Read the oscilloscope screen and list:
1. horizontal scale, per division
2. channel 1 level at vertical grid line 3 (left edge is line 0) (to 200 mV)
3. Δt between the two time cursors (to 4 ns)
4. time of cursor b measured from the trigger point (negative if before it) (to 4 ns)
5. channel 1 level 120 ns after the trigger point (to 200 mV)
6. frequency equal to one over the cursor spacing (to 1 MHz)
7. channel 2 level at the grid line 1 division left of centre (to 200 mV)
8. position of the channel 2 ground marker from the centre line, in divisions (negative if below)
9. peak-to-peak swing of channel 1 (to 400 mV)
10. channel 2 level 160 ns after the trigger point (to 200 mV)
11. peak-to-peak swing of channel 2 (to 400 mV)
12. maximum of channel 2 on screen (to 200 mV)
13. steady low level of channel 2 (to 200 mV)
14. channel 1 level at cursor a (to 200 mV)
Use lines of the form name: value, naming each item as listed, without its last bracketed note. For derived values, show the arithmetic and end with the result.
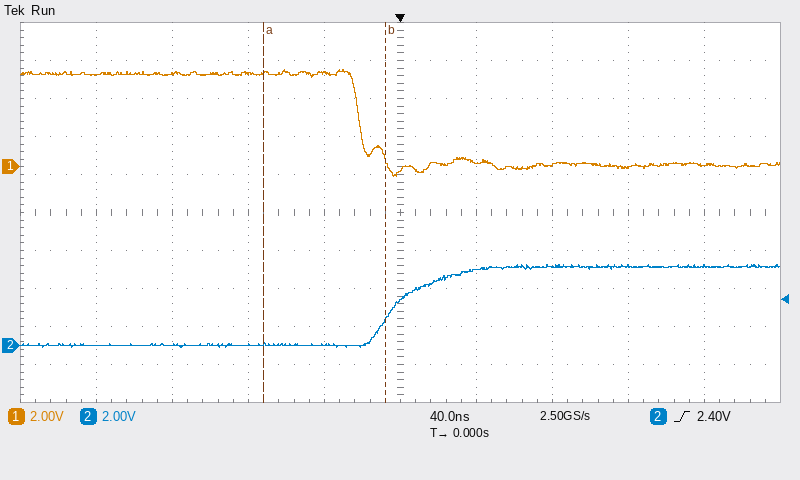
horizontal scale, per division: 40 ns
channel 1 level at vertical grid line 3 (left edge is line 0): 5.0 V
Δt between the two time cursors: 64 ns
time of cursor b measured from the trigger point (negative if before it): -8 ns
channel 1 level 120 ns after the trigger point: 0.0 V
frequency equal to one over the cursor spacing: 1 / 64 ns ≈ 16 MHz
channel 2 level at the grid line 1 division left of centre: 0.0 V
position of the channel 2 ground marker from the centre line, in divisions: -3.5 div
peak-to-peak swing of channel 1: 5.6 V
channel 2 level 160 ns after the trigger point: 4.2 V
peak-to-peak swing of channel 2: 4.4 V
maximum of channel 2 on screen: 4.2 V
steady low level of channel 2: 0.0 V
channel 1 level at cursor a: 5.0 V
